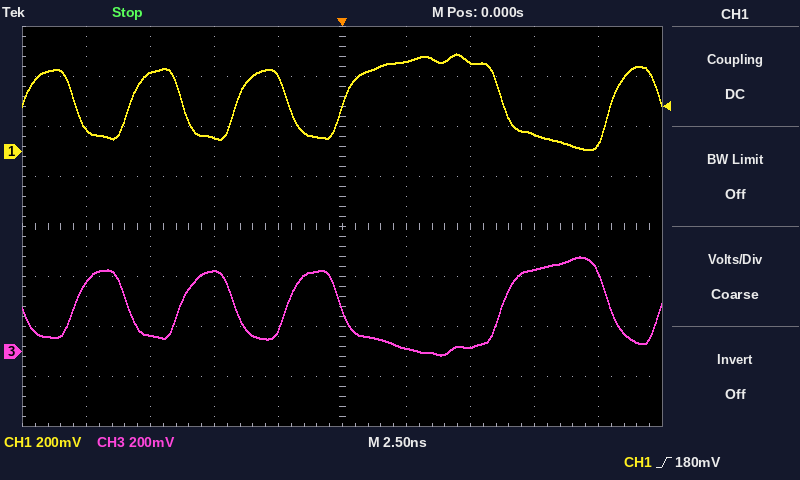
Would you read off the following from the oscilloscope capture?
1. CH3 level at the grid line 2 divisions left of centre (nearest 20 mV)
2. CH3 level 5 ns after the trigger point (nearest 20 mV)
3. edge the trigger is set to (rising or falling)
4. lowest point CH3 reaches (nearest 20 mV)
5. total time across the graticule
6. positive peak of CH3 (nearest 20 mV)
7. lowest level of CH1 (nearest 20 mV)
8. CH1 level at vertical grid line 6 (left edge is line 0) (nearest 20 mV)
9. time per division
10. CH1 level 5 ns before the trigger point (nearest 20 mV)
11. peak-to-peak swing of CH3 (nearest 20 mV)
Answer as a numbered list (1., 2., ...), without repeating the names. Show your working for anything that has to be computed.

1. 320 mV
2. 20 mV
3. rising
4. -20 mV
5. 25 ns
6. 380 mV
7. 0 mV
8. 360 mV
9. 2.5 ns
10. 60 mV
11. 380 mV − (-20 mV) = 400 mV
